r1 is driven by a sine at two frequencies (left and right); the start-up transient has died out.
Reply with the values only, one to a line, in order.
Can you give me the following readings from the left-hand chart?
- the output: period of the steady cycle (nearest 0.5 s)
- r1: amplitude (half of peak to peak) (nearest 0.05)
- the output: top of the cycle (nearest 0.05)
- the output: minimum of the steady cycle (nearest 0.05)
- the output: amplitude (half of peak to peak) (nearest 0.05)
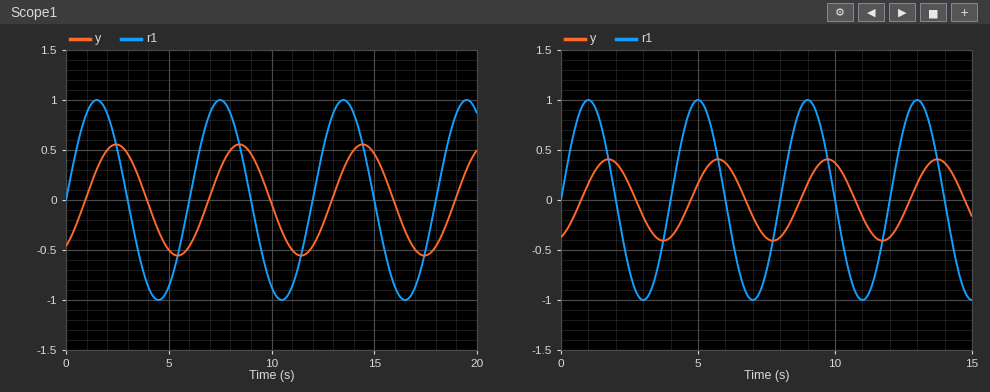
6.0 s
1.00
0.55
-0.55
0.55
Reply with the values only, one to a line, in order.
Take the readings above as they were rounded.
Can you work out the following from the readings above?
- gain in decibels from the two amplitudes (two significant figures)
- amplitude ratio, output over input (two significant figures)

-5.2 dB
0.55
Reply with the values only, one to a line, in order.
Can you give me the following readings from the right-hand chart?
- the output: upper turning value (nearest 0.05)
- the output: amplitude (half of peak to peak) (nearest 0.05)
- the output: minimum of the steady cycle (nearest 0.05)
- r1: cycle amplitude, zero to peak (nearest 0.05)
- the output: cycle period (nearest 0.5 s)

0.40
0.40
-0.40
1.00
4.0 s
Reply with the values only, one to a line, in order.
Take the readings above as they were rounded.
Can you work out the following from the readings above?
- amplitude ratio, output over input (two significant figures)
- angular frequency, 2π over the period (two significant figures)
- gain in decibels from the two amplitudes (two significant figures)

0.40
1.6 rad/s
-8.0 dB
